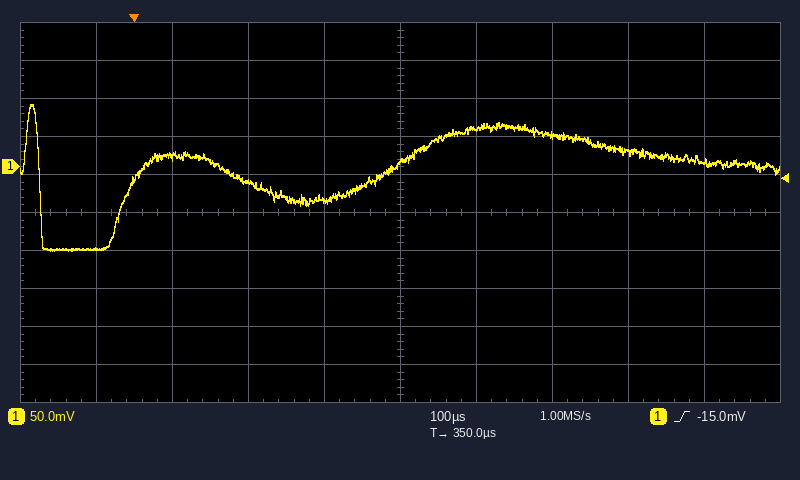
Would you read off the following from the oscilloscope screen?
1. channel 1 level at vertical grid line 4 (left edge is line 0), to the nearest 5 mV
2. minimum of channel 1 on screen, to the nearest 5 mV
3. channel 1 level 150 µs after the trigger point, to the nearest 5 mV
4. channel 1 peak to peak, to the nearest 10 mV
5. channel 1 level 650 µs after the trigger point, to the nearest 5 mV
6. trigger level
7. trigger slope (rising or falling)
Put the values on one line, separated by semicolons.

-45 mV; -110 mV; -20 mV; 190 mV; 20 mV; -15.0 mV; rising
